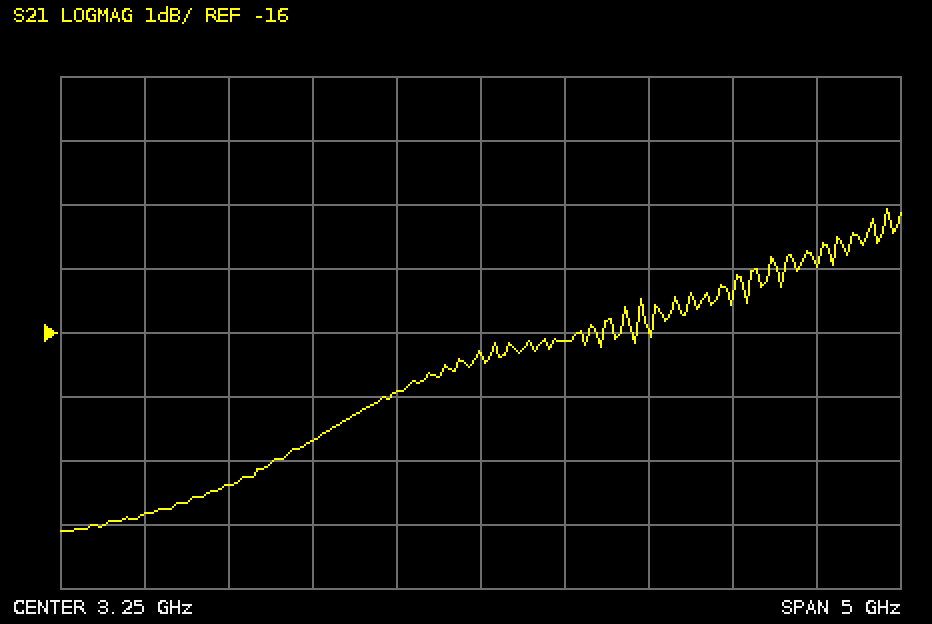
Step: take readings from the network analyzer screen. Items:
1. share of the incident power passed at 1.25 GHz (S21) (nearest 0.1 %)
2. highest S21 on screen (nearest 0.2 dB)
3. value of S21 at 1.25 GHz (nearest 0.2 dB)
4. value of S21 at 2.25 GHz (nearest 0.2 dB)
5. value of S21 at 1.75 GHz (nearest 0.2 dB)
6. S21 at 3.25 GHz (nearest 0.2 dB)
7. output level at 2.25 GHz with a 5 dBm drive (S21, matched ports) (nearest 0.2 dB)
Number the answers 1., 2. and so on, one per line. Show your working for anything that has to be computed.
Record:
1. 10^(-18.8/10) ≈ 1.3 %
2. -14.0 dB
3. -18.8 dB
4. -17.6 dB
5. -18.4 dB
6. -16.4 dB
7. 5 dBm + (-17.6 dB) = -12.6 dBm
